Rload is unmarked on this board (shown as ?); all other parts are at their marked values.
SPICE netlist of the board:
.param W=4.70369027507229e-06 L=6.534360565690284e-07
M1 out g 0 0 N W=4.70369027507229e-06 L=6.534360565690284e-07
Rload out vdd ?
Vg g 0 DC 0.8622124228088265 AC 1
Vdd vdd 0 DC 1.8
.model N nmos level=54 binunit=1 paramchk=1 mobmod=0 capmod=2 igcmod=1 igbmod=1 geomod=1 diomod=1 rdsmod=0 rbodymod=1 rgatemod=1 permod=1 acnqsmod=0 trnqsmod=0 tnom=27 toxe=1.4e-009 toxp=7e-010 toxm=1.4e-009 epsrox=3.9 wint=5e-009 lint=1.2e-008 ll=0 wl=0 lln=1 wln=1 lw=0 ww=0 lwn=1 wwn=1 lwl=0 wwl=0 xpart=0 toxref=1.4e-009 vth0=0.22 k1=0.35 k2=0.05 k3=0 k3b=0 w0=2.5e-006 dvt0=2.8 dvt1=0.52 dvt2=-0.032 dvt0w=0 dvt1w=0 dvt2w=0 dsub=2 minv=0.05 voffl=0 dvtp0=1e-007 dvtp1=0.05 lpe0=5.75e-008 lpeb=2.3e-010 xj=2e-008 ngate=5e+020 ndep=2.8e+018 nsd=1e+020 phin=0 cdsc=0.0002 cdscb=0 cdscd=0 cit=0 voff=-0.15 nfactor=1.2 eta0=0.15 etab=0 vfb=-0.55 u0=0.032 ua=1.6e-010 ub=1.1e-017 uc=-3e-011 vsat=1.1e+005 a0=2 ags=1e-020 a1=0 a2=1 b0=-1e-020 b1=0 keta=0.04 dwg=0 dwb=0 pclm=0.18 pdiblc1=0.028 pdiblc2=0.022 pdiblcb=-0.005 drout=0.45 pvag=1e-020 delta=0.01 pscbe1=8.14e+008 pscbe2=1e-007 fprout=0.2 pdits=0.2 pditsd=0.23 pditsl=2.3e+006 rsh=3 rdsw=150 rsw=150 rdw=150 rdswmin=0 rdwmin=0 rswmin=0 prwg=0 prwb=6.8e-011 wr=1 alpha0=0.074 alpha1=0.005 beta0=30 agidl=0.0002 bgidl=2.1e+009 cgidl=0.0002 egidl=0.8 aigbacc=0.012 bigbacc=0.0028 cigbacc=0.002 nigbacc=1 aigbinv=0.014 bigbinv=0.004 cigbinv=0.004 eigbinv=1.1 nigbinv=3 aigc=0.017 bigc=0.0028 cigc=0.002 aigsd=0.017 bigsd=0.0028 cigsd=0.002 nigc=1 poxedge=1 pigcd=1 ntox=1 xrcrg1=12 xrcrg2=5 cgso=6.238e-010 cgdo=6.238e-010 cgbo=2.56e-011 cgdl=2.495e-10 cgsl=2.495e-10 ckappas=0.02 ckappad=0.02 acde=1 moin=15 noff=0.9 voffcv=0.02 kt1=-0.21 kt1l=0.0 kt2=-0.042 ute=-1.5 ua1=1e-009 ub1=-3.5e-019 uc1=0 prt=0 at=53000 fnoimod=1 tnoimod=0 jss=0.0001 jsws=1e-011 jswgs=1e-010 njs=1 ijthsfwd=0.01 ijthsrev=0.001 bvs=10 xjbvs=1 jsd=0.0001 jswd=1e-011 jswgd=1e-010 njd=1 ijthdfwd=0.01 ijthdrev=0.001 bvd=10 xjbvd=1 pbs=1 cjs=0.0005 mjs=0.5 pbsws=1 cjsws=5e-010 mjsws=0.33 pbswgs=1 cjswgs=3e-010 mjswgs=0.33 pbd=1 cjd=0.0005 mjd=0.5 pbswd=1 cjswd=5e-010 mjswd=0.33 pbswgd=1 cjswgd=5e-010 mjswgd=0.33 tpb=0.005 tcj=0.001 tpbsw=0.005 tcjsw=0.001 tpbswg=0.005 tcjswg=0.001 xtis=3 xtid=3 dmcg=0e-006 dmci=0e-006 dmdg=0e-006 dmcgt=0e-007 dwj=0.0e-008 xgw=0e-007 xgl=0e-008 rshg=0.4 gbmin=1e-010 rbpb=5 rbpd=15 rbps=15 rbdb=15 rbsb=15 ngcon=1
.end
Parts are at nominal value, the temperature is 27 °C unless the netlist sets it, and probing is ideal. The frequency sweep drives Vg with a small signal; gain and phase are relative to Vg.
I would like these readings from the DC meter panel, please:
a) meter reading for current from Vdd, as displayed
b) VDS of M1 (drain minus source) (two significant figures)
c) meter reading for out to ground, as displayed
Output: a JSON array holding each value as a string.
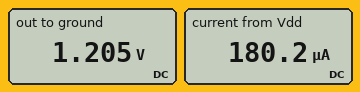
["180.2 µA", "1.2 V", "1.205 V"]
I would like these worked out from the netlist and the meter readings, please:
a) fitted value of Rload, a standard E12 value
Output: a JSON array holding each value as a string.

["3.3 kΩ"]
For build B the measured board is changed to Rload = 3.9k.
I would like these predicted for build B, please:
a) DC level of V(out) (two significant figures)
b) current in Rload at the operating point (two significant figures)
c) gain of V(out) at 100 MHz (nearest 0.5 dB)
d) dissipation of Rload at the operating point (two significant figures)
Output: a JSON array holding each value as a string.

["1.1 V", "180 µA", "0 dB", "120 µW"]
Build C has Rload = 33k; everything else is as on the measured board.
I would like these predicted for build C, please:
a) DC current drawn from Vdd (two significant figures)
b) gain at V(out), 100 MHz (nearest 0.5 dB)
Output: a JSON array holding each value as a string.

["52 µA", "-23.0 dB"]
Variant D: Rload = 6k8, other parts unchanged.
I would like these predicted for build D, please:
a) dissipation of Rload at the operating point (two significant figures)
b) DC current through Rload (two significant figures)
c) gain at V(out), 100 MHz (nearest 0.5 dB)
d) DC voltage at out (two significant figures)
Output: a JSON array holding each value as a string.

["190 µW", "170 µA", "4.0 dB", "650 mV"]
